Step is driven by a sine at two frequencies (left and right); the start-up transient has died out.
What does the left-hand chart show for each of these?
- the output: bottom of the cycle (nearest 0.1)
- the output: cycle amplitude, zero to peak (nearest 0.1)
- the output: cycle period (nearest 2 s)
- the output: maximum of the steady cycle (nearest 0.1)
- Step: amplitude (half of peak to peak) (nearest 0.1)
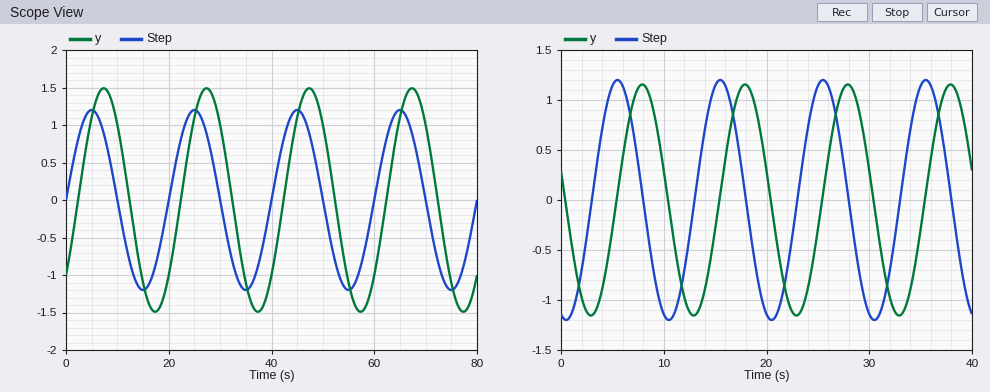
-1.5
1.5
20 s
1.5
1.2
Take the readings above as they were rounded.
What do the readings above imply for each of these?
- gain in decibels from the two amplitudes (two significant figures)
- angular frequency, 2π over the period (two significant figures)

1.9 dB
0.31 rad/s
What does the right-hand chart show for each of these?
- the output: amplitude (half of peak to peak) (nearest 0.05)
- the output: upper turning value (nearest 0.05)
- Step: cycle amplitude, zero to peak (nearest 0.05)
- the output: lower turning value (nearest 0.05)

1.15
1.15
1.20
-1.15
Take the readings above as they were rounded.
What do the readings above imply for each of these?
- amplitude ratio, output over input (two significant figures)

0.96
